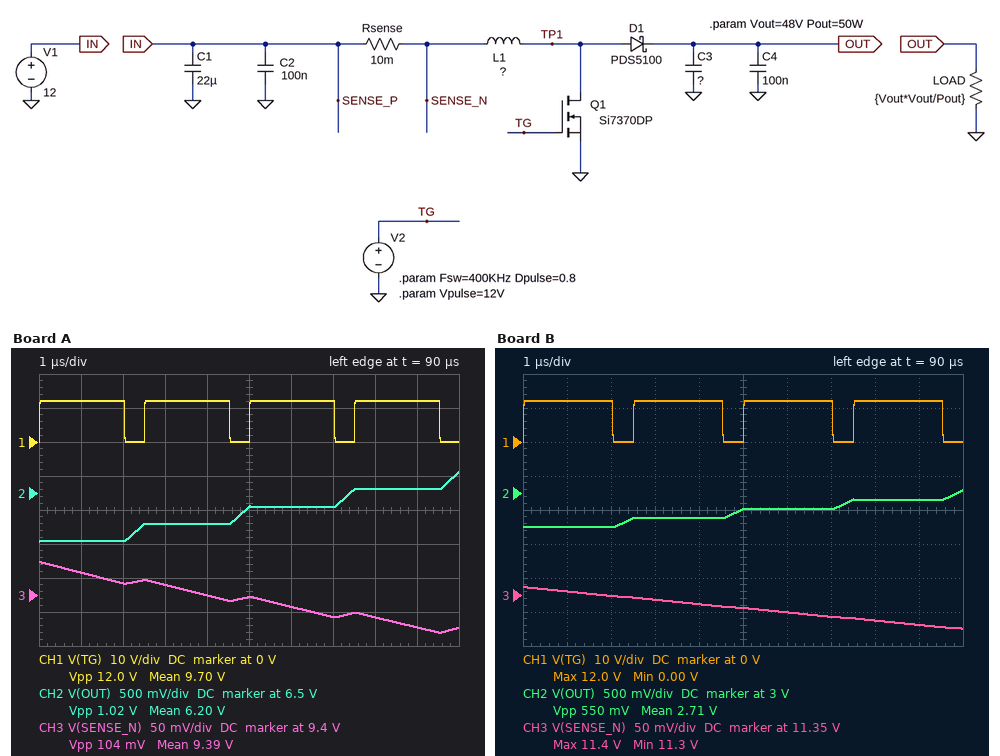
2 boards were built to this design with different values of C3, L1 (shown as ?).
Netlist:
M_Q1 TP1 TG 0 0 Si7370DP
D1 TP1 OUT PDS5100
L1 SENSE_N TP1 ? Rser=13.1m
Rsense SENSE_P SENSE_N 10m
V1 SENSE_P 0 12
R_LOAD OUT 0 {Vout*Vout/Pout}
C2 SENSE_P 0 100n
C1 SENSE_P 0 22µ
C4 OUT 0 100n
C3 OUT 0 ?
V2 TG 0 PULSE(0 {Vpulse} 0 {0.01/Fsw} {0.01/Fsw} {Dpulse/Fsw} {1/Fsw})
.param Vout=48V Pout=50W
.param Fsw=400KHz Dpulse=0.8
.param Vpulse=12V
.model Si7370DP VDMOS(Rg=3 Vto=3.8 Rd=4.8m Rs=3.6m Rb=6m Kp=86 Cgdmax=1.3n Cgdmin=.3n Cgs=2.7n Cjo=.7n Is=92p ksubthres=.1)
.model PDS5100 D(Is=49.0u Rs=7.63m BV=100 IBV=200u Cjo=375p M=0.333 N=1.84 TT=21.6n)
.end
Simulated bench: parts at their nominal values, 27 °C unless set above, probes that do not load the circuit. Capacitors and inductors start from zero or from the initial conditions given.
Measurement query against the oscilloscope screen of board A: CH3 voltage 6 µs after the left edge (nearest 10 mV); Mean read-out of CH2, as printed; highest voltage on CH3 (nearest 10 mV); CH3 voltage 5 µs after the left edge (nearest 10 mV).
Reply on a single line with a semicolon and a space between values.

9.38 V; 6.20 V; 9.45 V; 9.40 V
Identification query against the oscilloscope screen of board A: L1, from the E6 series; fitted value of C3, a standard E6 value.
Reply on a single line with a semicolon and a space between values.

2.2 µH; 470 µF
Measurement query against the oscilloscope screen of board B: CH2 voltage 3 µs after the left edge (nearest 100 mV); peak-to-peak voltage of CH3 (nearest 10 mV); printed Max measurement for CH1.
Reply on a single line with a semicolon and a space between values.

2.6 V; 60 mV; 12.0 V
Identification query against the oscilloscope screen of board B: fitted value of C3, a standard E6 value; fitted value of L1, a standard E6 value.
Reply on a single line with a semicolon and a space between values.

220 µF; 15 µH
